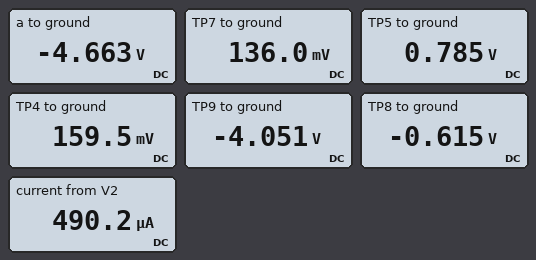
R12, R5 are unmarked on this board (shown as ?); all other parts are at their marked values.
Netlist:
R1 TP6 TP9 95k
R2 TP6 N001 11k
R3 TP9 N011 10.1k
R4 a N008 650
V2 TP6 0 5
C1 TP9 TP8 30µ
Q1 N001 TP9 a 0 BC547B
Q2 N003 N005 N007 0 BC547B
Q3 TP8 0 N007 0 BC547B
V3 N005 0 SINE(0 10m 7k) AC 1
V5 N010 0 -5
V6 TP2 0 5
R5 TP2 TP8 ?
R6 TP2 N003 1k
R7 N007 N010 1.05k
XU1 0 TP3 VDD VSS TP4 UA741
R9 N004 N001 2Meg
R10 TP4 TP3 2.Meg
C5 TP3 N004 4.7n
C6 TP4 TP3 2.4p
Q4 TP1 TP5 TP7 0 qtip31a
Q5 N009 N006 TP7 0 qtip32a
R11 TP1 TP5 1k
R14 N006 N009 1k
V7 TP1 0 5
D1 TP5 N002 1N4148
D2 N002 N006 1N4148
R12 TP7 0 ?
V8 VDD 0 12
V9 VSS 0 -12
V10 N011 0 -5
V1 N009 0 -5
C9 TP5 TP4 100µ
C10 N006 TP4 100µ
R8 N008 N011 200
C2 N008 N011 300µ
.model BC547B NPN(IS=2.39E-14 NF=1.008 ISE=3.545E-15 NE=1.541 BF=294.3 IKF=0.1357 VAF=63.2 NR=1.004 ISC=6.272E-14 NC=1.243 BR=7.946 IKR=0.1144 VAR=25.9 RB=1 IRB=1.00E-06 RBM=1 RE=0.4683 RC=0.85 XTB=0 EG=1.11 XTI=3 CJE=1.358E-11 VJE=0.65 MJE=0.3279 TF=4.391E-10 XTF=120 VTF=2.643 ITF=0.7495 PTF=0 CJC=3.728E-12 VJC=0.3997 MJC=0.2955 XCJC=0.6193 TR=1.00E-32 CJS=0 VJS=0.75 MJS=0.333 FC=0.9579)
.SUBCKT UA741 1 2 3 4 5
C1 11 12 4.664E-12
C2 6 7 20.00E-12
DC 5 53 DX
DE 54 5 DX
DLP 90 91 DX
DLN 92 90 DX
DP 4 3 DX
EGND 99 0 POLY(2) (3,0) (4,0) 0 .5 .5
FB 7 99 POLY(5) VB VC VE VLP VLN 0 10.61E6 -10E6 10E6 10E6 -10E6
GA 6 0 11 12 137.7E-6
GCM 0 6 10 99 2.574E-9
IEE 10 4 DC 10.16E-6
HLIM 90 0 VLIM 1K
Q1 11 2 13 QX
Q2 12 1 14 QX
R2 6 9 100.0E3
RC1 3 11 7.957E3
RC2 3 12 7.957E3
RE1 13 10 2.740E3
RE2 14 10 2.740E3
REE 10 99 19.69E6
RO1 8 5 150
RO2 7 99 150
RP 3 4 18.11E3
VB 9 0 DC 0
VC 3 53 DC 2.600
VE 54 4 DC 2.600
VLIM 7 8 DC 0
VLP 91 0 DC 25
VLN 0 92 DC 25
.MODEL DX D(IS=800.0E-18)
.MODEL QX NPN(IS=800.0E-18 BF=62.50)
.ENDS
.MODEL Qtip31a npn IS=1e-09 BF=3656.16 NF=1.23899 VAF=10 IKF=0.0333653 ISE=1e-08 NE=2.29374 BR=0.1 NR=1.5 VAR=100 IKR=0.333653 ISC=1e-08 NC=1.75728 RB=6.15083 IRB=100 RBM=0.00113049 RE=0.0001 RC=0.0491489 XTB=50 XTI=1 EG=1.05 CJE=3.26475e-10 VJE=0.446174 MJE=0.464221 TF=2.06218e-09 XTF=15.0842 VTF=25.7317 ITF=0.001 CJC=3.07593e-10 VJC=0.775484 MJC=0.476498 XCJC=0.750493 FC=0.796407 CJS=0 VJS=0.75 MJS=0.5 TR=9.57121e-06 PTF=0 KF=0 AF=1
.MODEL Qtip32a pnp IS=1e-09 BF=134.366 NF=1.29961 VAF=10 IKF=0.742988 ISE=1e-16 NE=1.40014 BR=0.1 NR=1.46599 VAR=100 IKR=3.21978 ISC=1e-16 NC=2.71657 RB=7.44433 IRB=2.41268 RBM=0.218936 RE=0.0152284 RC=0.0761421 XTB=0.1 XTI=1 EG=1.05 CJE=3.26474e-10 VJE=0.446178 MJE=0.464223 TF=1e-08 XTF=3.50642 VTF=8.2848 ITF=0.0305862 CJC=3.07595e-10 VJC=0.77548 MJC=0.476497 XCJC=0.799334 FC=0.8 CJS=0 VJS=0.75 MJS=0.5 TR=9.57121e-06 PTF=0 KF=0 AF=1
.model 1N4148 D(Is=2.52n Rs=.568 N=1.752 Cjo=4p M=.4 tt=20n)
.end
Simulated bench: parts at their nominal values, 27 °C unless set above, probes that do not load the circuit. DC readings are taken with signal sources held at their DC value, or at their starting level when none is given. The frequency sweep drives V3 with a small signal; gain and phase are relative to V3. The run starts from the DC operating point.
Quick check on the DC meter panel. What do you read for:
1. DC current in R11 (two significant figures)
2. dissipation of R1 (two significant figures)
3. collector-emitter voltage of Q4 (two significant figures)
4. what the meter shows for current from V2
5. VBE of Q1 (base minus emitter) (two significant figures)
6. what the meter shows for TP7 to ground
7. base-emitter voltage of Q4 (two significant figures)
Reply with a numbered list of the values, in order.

1. 4.2 mA
2. 860 µW
3. 4.9 V
4. 490.2 µA
5. 610 mV
6. 136.0 mV
7. 650 mV
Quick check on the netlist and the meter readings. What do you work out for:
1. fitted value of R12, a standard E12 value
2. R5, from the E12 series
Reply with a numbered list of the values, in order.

1. 18 Ω
2. 3.3 kΩ
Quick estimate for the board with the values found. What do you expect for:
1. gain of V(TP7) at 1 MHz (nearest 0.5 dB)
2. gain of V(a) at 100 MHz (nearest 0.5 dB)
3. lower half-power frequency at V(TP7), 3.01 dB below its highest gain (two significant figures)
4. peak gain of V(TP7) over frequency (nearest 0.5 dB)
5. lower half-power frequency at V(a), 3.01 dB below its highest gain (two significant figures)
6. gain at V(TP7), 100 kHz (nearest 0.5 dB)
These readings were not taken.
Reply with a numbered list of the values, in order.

1. -1.5 dB
2. 0 dB
3. 17 Hz
4. 34.0 dB
5. 570 mHz
6. 23.5 dB
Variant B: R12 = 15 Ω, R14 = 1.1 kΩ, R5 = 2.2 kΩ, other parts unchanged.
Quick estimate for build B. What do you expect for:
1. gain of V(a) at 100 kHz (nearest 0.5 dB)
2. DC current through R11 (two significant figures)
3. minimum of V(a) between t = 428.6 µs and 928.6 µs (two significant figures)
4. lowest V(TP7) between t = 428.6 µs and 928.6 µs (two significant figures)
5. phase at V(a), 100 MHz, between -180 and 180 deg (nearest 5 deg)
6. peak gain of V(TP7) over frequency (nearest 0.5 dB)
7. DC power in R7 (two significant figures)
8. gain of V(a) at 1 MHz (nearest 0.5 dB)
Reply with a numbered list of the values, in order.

1. 35.0 dB
2. 4.1 mA
3. -4.9 V
4. -4.0 V
5. -45 deg
6. 59.5 dB
7. 18 mW
8. 34.0 dB
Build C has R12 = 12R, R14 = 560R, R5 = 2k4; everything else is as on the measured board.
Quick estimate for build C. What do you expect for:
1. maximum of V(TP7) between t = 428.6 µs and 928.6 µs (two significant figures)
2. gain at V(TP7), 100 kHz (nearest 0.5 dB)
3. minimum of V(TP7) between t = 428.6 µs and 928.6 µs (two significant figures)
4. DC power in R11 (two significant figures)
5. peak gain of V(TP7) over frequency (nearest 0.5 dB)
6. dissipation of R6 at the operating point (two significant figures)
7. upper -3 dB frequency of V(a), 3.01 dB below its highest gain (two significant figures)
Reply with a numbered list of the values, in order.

1. 4.0 V
2. 49.0 dB
3. -4.8 V
4. 27 mW
5. 60.0 dB
6. 4.4 mW
7. 2.0 MHz
